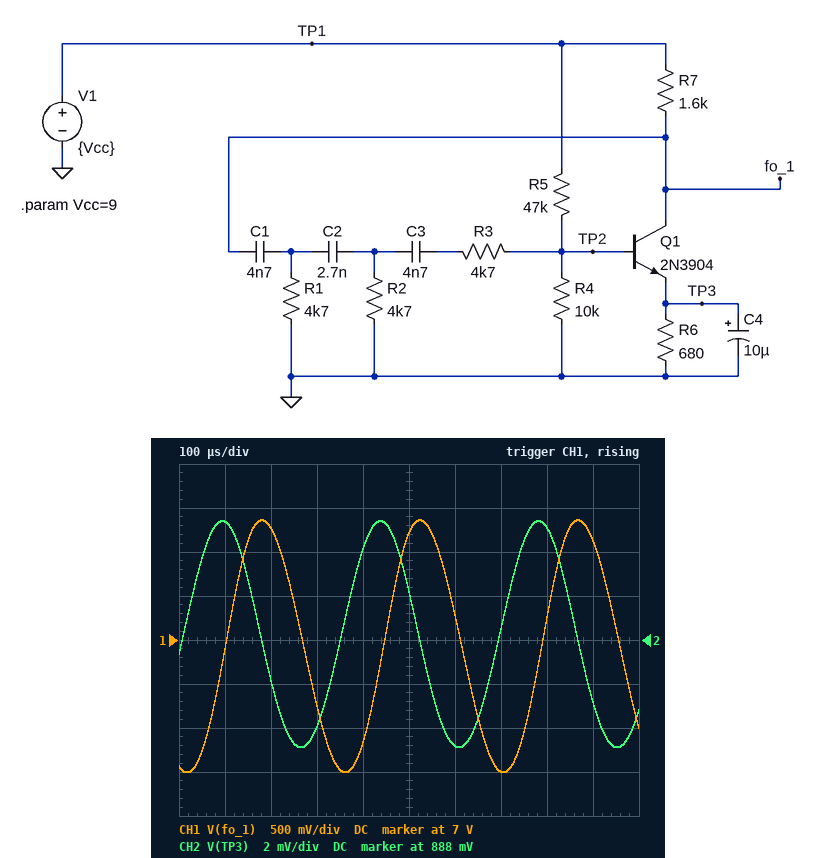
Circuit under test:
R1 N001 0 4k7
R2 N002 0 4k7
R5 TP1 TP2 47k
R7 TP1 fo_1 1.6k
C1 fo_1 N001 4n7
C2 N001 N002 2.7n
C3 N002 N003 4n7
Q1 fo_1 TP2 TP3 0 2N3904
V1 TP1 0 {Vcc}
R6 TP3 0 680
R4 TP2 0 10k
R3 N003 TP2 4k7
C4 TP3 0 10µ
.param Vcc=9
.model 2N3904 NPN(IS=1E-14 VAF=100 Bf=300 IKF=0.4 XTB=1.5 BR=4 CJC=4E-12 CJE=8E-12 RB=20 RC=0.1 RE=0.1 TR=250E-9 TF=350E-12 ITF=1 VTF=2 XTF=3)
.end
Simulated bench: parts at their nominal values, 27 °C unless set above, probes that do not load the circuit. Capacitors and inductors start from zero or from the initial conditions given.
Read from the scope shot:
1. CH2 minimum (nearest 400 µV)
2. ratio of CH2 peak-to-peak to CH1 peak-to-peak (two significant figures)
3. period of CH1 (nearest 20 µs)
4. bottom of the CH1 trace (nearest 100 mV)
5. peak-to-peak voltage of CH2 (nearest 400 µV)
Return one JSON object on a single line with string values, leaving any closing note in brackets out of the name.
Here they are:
{"CH2 minimum": "883.2 mV", "ratio of CH2 peak-to-peak to CH1 peak-to-peak": "0.0036", "period of CH1": "340 µs", "bottom of the CH1 trace": "5.5 V", "peak-to-peak voltage of CH2": "10.4 mV"}
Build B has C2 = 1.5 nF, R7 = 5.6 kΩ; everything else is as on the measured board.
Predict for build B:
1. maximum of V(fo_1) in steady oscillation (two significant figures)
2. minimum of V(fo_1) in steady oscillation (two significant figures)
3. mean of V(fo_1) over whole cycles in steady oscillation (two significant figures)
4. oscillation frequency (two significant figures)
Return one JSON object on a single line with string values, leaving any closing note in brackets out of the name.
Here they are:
{"maximum of V(fo_1) in steady oscillation": "2.5 V", "minimum of V(fo_1) in steady oscillation": "990 mV", "mean of V(fo_1) over whole cycles in steady oscillation": "1.8 V", "oscillation frequency": "2.7 kHz"}
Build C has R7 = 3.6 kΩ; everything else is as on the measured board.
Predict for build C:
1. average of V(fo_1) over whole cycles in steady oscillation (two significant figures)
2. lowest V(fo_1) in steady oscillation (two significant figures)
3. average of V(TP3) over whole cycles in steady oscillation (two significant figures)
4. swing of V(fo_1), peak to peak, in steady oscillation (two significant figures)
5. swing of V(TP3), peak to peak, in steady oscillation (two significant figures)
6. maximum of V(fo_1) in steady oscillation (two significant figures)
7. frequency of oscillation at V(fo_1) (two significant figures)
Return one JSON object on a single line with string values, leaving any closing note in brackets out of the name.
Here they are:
{"average of V(fo_1) over whole cycles in steady oscillation": "4.4 V", "lowest V(fo_1) in steady oscillation": "950 mV", "average of V(TP3) over whole cycles in steady oscillation": "870 mV", "swing of V(fo_1), peak to peak, in steady oscillation": "7.0 V", "swing of V(TP3), peak to peak, in steady oscillation": "14 mV", "maximum of V(fo_1) in steady oscillation": "7.9 V", "frequency of oscillation at V(fo_1)": "2.5 kHz"}
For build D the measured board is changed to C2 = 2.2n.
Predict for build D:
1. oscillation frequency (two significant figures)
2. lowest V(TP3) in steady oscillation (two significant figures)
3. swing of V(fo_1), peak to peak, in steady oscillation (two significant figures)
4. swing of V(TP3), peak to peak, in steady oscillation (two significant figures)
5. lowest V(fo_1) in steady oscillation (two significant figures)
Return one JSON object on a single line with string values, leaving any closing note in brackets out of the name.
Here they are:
{"oscillation frequency": "3.1 kHz", "lowest V(TP3) in steady oscillation": "880 mV", "swing of V(fo_1), peak to peak, in steady oscillation": "2.0 V", "swing of V(TP3), peak to peak, in steady oscillation": "6.9 mV", "lowest V(fo_1) in steady oscillation": "5.9 V"}
